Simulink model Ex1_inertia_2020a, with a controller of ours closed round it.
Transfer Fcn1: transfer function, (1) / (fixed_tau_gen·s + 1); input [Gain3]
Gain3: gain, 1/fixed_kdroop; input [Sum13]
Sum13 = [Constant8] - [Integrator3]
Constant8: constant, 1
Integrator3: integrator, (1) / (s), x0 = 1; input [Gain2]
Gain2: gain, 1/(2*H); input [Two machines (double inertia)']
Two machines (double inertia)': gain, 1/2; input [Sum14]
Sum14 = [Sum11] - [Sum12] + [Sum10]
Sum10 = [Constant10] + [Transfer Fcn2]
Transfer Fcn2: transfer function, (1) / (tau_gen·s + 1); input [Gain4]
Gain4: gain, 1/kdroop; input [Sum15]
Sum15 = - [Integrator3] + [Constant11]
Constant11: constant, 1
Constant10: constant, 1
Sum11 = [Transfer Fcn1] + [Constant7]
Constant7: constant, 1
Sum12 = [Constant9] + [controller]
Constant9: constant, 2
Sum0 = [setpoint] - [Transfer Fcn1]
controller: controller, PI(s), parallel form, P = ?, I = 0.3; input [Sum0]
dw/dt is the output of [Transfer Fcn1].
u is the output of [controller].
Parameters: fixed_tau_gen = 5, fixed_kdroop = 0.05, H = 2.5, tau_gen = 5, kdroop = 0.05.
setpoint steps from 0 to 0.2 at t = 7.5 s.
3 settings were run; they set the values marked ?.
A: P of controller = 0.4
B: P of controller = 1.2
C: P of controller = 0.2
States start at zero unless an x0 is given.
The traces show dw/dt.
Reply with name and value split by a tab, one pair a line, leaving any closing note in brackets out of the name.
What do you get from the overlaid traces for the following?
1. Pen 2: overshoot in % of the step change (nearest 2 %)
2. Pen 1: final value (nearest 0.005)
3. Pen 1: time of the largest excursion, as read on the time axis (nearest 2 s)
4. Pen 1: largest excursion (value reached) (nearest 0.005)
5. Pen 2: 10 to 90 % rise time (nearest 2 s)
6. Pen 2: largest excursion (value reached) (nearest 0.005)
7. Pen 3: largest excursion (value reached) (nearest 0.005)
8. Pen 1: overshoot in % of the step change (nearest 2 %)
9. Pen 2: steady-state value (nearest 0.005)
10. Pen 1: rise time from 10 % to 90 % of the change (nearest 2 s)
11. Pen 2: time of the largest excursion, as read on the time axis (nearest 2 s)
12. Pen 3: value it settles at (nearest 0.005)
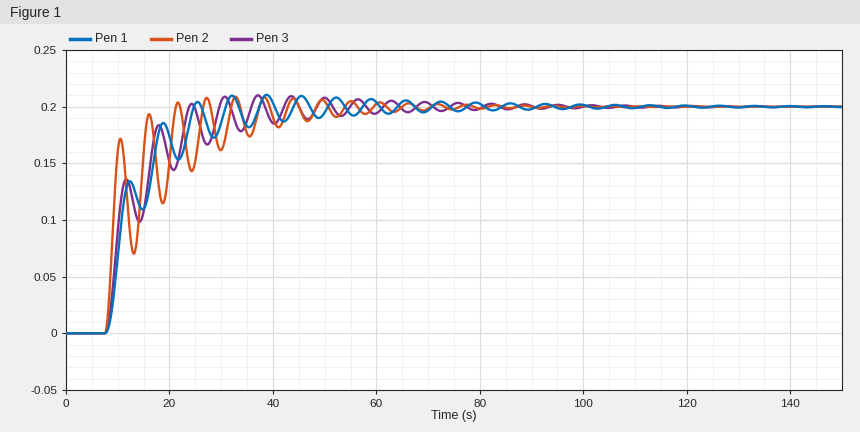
Pen 2: overshoot in % of the step change	4 %
Pen 1: final value	0.200
Pen 1: time of the largest excursion, as read on the time axis	38 s
Pen 1: largest excursion (value reached)	0.210
Pen 2: 10 to 90 % rise time	8 s
Pen 2: largest excursion (value reached)	0.210
Pen 3: largest excursion (value reached)	0.210
Pen 1: overshoot in % of the step change	6 %
Pen 2: steady-state value	0.200
Pen 1: rise time from 10 % to 90 % of the change	10 s
Pen 2: time of the largest excursion, as read on the time axis	32 s
Pen 3: value it settles at	0.200
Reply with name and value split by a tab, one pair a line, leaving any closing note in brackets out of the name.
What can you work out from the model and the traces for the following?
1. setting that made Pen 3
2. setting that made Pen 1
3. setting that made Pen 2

setting that made Pen 3	A
setting that made Pen 1	C
setting that made Pen 2	B
